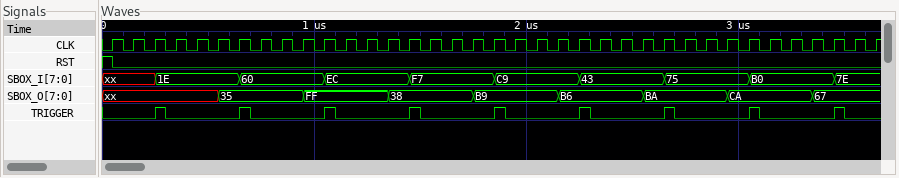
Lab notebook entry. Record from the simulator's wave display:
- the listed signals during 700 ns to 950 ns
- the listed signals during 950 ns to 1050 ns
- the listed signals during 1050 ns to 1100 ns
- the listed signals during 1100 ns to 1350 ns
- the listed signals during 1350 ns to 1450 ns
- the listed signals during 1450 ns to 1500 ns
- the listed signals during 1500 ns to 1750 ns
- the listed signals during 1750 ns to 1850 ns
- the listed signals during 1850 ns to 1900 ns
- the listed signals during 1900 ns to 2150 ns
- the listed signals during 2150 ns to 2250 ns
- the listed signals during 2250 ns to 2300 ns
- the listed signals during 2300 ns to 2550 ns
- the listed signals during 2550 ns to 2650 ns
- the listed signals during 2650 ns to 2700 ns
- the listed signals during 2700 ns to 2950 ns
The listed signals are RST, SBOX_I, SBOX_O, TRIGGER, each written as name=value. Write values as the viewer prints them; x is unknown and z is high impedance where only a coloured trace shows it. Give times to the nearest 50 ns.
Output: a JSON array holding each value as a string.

["RST=0, SBOX_I=60, SBOX_O=35, TRIGGER=0", "RST=0, SBOX_I=60, SBOX_O=FF, TRIGGER=0", "RST=0, SBOX_I=EC, SBOX_O=FF, TRIGGER=1", "RST=0, SBOX_I=EC, SBOX_O=FF, TRIGGER=0", "RST=0, SBOX_I=EC, SBOX_O=38, TRIGGER=0", "RST=0, SBOX_I=F7, SBOX_O=38, TRIGGER=1", "RST=0, SBOX_I=F7, SBOX_O=38, TRIGGER=0", "RST=0, SBOX_I=F7, SBOX_O=B9, TRIGGER=0", "RST=0, SBOX_I=C9, SBOX_O=B9, TRIGGER=1", "RST=0, SBOX_I=C9, SBOX_O=B9, TRIGGER=0", "RST=0, SBOX_I=C9, SBOX_O=B6, TRIGGER=0", "RST=0, SBOX_I=43, SBOX_O=B6, TRIGGER=1", "RST=0, SBOX_I=43, SBOX_O=B6, TRIGGER=0", "RST=0, SBOX_I=43, SBOX_O=BA, TRIGGER=0", "RST=0, SBOX_I=75, SBOX_O=BA, TRIGGER=1", "RST=0, SBOX_I=75, SBOX_O=BA, TRIGGER=0"]
